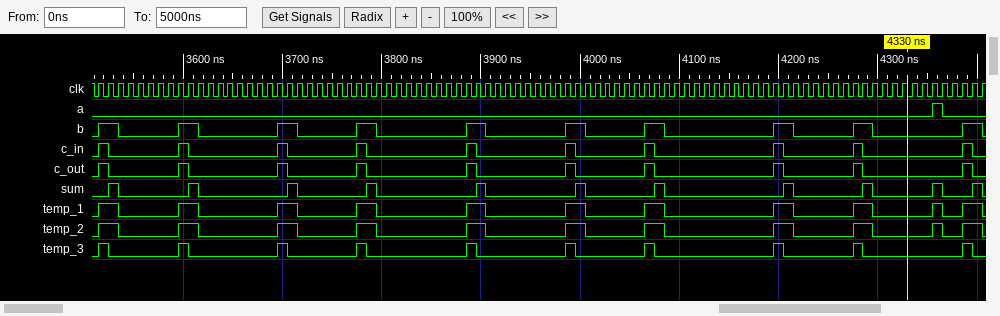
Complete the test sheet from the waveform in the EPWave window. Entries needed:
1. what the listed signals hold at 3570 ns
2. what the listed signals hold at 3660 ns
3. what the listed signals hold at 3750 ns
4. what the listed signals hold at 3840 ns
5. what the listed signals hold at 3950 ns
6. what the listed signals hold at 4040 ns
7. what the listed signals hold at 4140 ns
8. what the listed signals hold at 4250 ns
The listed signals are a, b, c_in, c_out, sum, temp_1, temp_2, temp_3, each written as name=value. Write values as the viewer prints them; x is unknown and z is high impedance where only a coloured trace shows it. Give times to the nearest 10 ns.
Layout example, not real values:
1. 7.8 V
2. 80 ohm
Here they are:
1. a=0, b=0, c_in=0, c_out=0, sum=0, temp_1=0, temp_2=0, temp_3=0
2. a=0, b=0, c_in=0, c_out=0, sum=0, temp_1=0, temp_2=0, temp_3=0
3. a=0, b=0, c_in=0, c_out=0, sum=0, temp_1=0, temp_2=0, temp_3=0
4. a=0, b=0, c_in=0, c_out=0, sum=0, temp_1=0, temp_2=0, temp_3=0
5. a=0, b=0, c_in=0, c_out=0, sum=0, temp_1=0, temp_2=0, temp_3=0
6. a=0, b=0, c_in=0, c_out=0, sum=0, temp_1=0, temp_2=0, temp_3=0
7. a=0, b=0, c_in=0, c_out=0, sum=0, temp_1=0, temp_2=0, temp_3=0
8. a=0, b=0, c_in=0, c_out=0, sum=0, temp_1=0, temp_2=0, temp_3=0
